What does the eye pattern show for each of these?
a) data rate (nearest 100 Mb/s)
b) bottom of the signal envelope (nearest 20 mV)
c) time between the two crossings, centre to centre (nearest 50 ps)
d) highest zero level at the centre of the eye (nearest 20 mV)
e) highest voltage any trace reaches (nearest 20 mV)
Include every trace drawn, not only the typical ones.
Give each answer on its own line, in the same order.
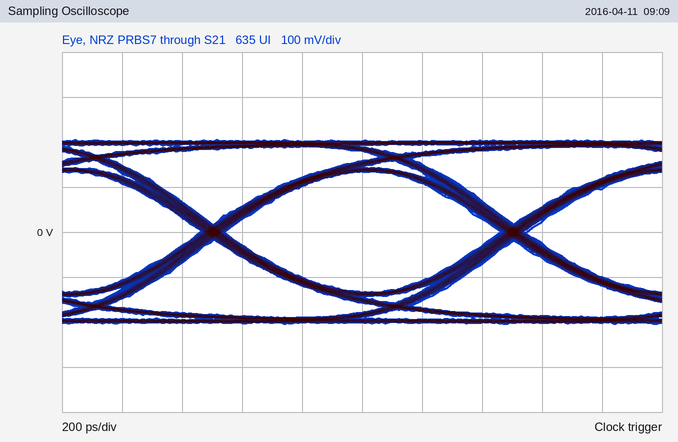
1.0 Gb/s
-200 mV
1.00 ns
-140 mV
200 mV
